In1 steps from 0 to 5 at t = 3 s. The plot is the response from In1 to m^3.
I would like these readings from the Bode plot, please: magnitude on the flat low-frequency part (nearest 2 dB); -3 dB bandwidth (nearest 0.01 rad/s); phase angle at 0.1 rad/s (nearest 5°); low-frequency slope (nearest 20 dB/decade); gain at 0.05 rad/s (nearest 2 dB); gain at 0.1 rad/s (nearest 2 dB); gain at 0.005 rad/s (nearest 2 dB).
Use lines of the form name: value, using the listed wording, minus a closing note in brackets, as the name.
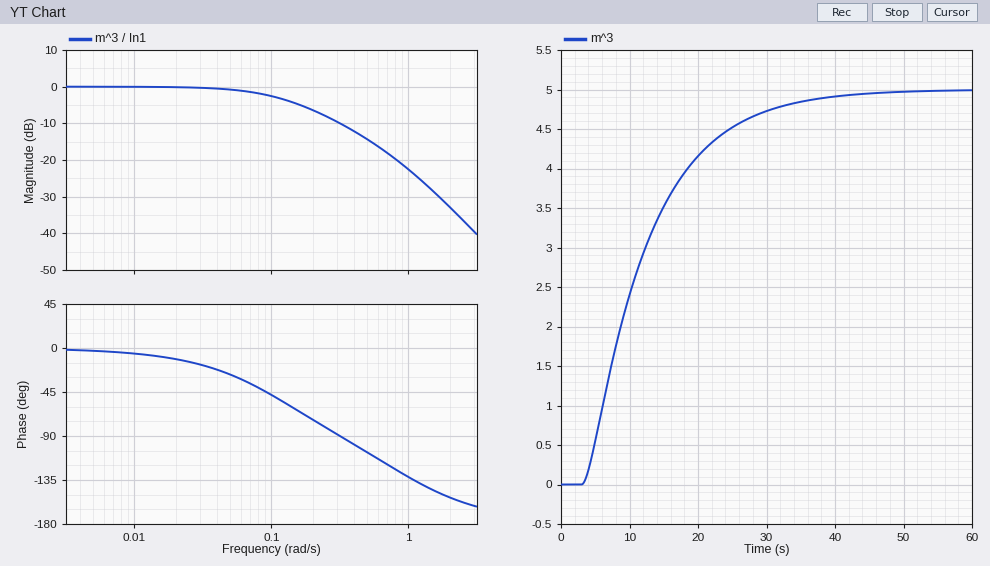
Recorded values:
magnitude on the flat low-frequency part: 0 dB
-3 dB bandwidth: 0.11 rad/s
phase angle at 0.1 rad/s: -50°
low-frequency slope: 0 dB/decade
gain at 0.05 rad/s: 0 dB
gain at 0.1 rad/s: -2 dB
gain at 0.005 rad/s: 0 dB
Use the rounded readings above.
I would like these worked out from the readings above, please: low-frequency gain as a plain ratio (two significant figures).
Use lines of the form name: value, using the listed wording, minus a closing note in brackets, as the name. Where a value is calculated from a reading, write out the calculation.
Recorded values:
low-frequency gain as a plain ratio: 10^(0 / 20) = 1.0
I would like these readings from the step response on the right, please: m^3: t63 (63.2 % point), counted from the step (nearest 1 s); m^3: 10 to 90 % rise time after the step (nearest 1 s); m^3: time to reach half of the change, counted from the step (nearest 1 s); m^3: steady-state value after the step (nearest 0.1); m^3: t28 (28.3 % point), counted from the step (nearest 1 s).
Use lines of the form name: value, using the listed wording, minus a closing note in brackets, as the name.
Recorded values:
m^3: t63 (63.2 % point), counted from the step: 10 s
m^3: 10 to 90 % rise time after the step: 20 s
m^3: time to reach half of the change, counted from the step: 7 s
m^3: steady-state value after the step: 5.0
m^3: t28 (28.3 % point), counted from the step: 4 s
